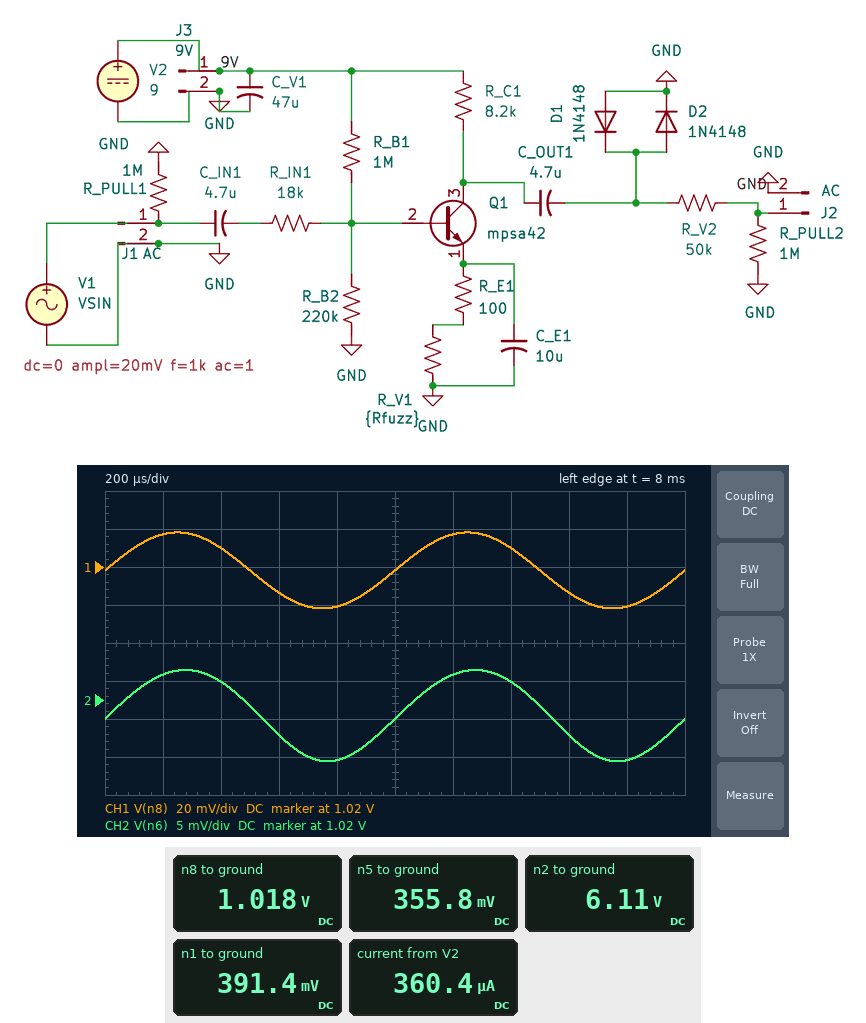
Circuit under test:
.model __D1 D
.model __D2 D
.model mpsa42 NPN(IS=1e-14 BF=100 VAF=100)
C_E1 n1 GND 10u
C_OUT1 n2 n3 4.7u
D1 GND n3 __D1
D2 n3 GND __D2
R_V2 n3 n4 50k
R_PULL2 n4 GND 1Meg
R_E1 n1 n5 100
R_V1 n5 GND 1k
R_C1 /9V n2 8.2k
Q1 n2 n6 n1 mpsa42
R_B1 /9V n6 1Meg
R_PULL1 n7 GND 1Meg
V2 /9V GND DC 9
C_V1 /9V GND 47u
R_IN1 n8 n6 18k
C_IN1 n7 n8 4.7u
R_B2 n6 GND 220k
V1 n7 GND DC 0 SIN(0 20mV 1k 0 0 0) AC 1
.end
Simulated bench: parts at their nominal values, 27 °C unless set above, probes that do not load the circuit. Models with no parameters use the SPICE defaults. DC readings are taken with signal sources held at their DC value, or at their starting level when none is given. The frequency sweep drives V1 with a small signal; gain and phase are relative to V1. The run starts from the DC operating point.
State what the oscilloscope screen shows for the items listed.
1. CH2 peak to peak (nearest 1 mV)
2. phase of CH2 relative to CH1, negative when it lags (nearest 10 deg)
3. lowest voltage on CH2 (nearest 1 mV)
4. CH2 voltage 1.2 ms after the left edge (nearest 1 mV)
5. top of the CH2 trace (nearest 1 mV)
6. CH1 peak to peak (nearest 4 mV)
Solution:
12 mV
-10 deg
1.012 V
1.023 V
1.024 V
40 mV
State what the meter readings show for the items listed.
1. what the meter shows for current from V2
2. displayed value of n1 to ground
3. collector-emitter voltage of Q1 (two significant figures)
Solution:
360.4 µA
391.4 mV
5.7 V
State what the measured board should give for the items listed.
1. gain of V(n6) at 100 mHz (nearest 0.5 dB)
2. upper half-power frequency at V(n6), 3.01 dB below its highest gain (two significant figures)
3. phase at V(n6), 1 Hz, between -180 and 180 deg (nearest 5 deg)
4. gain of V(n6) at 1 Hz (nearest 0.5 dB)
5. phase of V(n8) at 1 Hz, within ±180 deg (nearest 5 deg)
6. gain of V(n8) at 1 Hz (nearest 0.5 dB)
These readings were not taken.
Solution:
-13.5 dB
99 Hz
20 deg
-2.5 dB
20 deg
-0.5 dB
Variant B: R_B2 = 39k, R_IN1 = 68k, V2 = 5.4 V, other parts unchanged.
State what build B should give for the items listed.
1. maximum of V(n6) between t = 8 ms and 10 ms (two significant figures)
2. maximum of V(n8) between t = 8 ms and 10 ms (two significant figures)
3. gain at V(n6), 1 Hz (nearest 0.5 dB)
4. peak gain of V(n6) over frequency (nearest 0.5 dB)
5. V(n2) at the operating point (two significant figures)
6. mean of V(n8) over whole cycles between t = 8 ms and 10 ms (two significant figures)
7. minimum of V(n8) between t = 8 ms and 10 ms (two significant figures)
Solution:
210 mV
220 mV
-9.5 dB
-9.0 dB
5.4 V
200 mV
180 mV
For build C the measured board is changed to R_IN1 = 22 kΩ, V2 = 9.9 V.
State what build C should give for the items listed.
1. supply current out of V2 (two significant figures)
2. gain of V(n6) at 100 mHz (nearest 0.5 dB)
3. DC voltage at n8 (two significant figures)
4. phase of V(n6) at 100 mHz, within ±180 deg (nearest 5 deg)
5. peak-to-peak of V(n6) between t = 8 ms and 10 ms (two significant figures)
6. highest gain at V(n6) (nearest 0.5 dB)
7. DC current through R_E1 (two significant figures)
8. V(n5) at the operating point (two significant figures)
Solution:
420 µA
-14.0 dB
1.1 V
75 deg
9.4 mV
-2.5 dB
410 µA
410 mV
